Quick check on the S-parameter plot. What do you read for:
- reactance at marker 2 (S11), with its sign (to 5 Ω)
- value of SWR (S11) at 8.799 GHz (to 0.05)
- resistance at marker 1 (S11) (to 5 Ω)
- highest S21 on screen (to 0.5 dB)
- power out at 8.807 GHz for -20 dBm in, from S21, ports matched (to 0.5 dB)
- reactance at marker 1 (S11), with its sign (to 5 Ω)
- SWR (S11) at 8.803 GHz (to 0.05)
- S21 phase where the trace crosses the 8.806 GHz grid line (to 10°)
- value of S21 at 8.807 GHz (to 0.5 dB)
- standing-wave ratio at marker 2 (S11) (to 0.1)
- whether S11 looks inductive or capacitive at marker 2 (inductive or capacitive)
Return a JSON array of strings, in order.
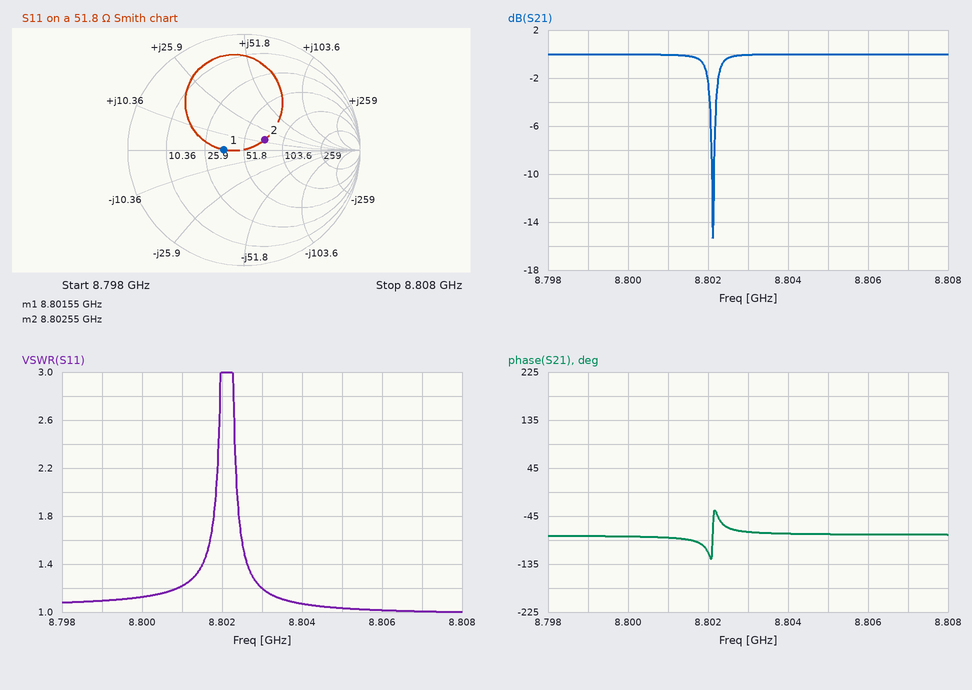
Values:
["+15 Ω", "1.10", "35 Ω", "0.0 dB", "-20.0 dBm", "0 Ω", "1.20", "-80°", "0.0 dB", "1.5", "inductive"]
